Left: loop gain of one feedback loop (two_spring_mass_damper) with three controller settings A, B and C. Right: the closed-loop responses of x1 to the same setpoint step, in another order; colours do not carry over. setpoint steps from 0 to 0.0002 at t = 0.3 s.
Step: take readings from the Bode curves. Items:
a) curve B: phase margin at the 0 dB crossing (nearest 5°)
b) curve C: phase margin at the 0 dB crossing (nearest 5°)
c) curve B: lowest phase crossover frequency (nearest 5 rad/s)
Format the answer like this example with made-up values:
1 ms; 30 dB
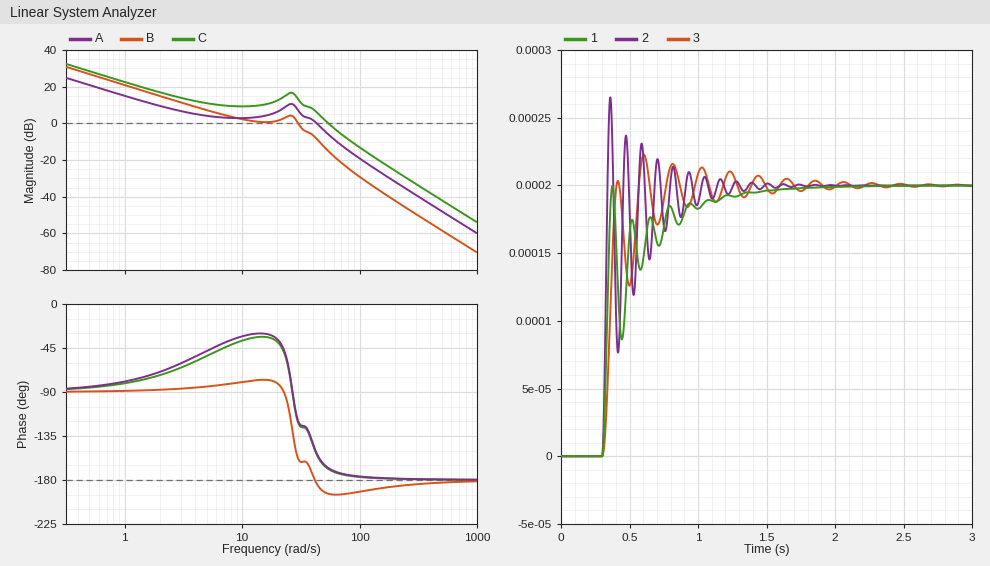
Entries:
20°; 10°; 40 rad/s
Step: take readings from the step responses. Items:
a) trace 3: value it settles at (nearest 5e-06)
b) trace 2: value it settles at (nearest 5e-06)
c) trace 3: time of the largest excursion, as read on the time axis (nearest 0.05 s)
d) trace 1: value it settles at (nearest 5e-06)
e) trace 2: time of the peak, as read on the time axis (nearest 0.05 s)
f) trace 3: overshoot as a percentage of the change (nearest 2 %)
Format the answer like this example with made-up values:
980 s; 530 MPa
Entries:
0.000200; 0.000200; 0.60 s; 0.000200; 0.35 s; 12 %
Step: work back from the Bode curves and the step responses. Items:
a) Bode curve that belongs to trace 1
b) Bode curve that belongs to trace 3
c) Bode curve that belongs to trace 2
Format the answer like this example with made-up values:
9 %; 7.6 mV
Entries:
A; B; C
